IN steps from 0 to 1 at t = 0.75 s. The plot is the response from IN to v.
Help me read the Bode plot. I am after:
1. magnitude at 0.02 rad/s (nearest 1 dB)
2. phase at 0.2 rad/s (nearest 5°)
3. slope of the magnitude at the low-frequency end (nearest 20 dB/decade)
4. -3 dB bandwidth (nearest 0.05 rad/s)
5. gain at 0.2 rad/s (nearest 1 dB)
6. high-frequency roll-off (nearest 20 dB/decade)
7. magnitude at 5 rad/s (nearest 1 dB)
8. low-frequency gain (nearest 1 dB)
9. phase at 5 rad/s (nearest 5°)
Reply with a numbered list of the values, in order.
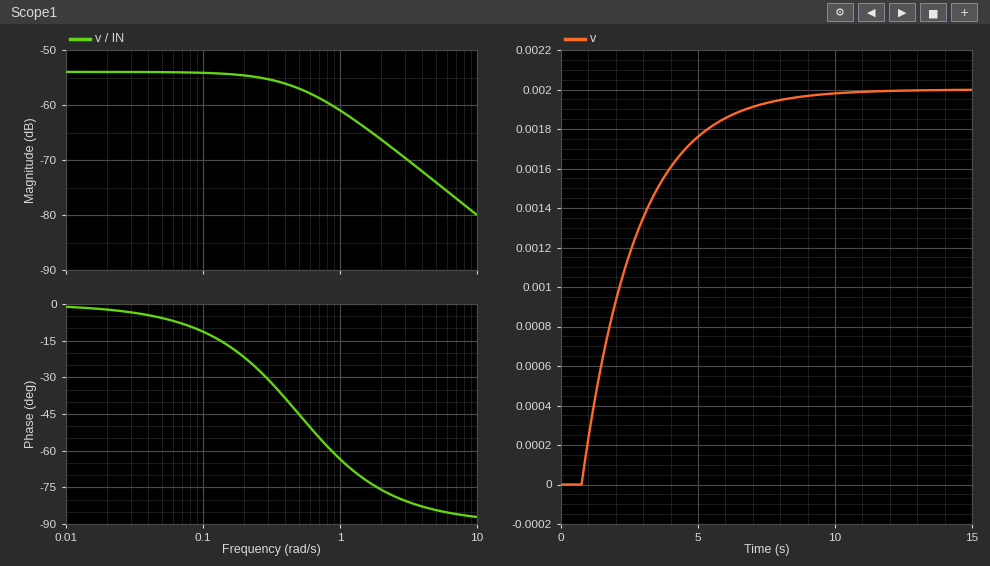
1. -54 dB
2. -20°
3. 0 dB/decade
4. 0.50 rad/s
5. -55 dB
6. -20 dB/decade
7. -74 dB
8. -54 dB
9. -85°
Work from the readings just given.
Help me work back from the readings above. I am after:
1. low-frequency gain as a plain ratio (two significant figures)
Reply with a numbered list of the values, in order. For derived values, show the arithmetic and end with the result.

1. 10^(-54 / 20) = 0.0020
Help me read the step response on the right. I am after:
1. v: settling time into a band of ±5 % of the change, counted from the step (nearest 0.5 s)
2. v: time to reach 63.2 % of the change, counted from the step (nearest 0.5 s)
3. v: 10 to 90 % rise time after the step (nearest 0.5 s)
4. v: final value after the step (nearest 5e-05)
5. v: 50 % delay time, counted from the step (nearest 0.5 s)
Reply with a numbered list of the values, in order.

1. 6.0 s
2. 2.0 s
3. 4.5 s
4. 0.00200
5. 1.5 s
